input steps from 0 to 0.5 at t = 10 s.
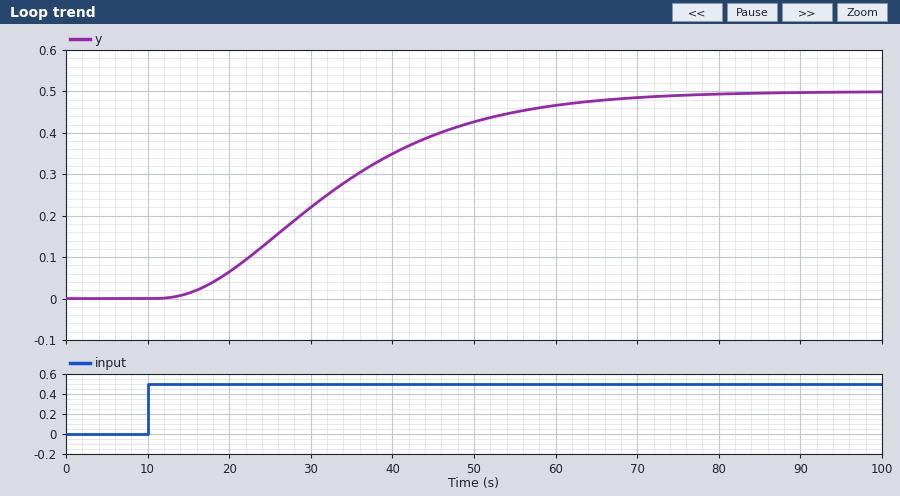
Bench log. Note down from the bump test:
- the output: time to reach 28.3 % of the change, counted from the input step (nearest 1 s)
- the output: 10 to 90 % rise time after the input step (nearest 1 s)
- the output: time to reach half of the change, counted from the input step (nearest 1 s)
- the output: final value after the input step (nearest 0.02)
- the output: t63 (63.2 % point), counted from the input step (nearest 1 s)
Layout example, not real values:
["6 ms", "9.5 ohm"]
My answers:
["15 s", "36 s", "22 s", "0.50", "27 s"]
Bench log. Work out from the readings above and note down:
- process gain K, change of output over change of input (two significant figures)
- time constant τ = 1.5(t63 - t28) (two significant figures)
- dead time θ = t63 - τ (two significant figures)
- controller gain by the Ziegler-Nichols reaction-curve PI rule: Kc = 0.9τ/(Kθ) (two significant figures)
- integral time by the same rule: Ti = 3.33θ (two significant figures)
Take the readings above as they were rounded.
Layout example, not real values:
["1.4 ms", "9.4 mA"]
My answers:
["1.0", "18 s", "9.0 s", "1.8", "30 s"]
